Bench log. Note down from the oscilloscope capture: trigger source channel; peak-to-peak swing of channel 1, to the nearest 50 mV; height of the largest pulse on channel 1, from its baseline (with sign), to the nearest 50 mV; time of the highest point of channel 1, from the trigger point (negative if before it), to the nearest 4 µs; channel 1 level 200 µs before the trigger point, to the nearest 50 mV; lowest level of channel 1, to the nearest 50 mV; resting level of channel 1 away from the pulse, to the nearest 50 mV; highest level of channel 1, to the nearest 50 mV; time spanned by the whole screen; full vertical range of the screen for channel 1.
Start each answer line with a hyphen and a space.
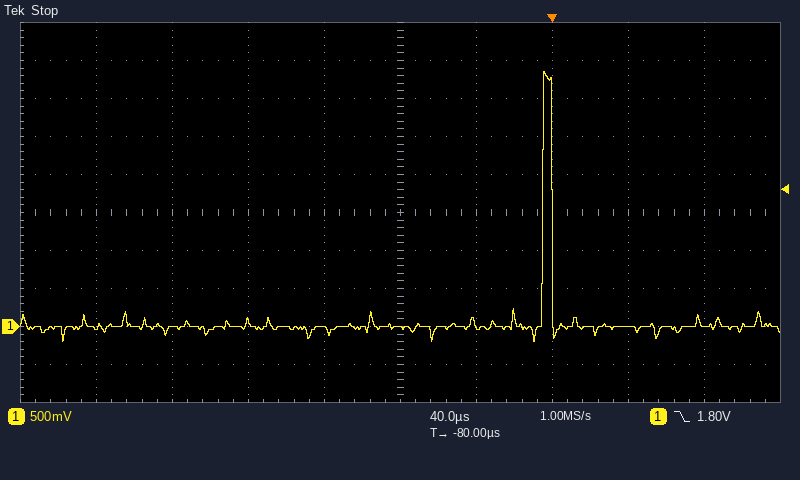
- channel 1
- 3.55 V
- +3.35 V
- -4 µs
- 0 mV
- -200 mV
- 0 mV
- 3.35 V
- 400 µs
- 5 V
